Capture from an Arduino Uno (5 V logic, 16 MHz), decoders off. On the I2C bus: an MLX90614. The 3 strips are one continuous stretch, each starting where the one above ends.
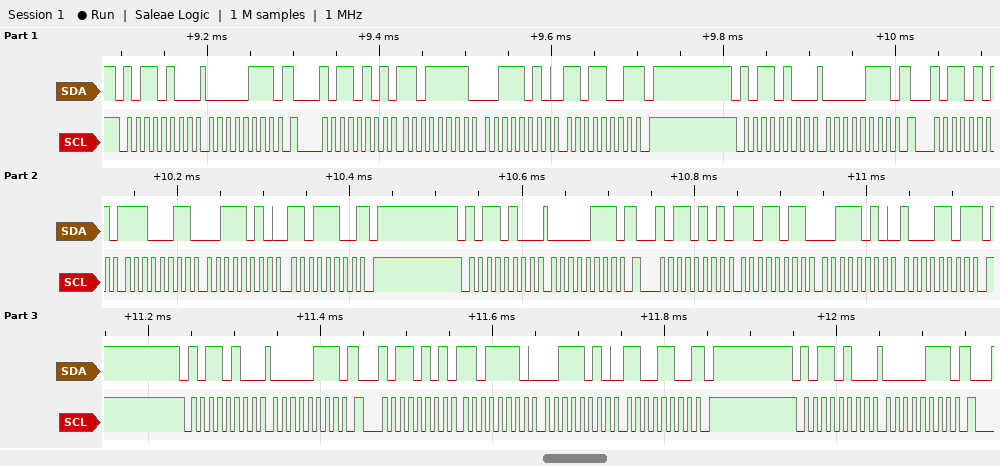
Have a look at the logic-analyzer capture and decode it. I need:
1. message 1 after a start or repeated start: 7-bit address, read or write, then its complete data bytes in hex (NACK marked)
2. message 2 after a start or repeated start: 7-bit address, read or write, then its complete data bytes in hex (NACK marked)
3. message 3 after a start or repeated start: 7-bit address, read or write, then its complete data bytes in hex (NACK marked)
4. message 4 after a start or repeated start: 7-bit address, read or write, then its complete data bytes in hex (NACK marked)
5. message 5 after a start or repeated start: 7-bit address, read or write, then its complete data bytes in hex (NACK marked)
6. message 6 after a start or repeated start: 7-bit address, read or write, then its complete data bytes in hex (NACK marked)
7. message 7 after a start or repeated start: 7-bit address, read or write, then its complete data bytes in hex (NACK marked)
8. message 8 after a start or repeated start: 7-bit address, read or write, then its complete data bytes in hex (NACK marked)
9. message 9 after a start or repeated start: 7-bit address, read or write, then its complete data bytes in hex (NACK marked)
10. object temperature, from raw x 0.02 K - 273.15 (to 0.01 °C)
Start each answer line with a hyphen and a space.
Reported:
- 0x5A write: 07
- 0x5A read: DF 3A D9 NACK
- 0x5A write: 07
- 0x5A read: E3 3A DC NACK
- 0x5A write: 07
- 0x5A read: DB 3A 8D NACK
- 0x5A write: 07
- 0x5A read: DE 3A CC NACK
- 0x5A write: 07
- 28.27 °C
